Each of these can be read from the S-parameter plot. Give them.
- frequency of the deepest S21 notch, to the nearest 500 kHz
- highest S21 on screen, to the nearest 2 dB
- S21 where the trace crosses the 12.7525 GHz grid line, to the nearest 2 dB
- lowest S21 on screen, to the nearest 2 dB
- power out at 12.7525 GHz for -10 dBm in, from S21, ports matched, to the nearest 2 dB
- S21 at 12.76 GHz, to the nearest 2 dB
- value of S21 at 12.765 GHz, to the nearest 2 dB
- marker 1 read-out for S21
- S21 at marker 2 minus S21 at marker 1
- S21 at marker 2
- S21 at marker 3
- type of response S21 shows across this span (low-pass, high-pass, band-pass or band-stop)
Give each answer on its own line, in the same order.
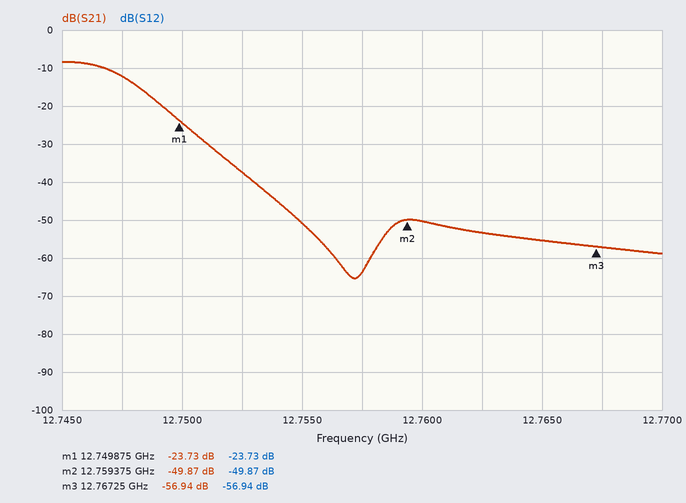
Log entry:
12.7570 GHz
-8 dB
-38 dB
-66 dB
-48 dBm
-50 dB
-56 dB
-23.73 dB
-26.14 dB
-49.87 dB
-56.94 dB
low-pass
